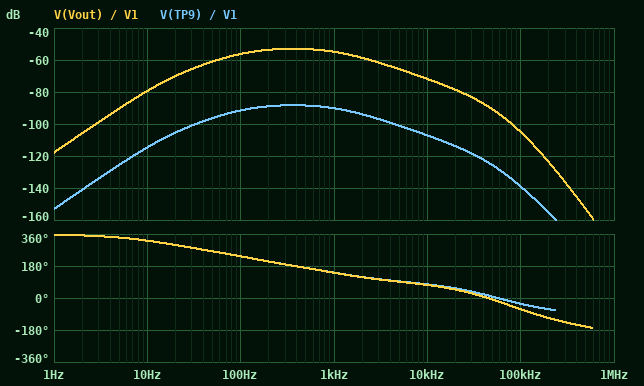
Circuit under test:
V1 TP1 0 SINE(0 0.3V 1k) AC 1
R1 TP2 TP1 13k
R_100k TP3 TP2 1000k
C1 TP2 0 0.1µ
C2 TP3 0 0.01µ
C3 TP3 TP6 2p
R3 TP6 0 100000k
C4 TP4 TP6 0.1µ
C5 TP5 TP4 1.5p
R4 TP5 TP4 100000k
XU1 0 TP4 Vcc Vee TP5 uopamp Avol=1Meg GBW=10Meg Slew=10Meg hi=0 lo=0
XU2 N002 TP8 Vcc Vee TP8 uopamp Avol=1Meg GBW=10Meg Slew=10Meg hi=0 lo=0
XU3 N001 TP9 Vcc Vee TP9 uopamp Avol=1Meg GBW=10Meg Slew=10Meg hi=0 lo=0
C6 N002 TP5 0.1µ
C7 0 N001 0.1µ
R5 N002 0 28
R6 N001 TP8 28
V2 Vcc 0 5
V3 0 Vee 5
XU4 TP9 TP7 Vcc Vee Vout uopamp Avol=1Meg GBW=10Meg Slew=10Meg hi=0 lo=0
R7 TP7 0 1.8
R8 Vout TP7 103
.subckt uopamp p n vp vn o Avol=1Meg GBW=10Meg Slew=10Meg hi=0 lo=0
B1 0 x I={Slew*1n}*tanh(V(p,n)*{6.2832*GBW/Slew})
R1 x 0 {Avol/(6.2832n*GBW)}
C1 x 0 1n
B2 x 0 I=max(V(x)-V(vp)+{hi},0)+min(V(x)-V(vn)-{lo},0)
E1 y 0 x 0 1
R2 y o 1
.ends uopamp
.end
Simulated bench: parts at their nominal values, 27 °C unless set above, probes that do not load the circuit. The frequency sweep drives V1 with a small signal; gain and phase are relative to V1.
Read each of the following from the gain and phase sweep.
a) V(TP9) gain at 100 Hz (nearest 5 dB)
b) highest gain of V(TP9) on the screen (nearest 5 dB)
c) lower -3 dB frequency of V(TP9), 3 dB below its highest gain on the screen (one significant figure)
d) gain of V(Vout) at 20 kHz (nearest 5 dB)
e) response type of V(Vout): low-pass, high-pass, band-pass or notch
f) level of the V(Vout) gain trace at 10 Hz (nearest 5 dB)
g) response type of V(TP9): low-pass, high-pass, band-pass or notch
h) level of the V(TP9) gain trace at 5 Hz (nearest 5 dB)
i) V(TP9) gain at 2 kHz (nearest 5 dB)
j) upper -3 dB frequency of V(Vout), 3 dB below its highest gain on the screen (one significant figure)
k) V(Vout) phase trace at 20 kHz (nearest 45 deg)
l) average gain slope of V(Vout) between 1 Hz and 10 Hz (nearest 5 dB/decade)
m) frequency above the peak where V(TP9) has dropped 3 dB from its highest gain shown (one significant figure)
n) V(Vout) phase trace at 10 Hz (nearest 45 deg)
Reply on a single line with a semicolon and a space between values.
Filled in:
-90 dB; -90 dB; 100 Hz; -80 dB; band-pass; -80 dB; band-pass; -125 dB; -95 dB; 1 kHz; 45 deg; 40 dB/decade; 1 kHz; 315 deg
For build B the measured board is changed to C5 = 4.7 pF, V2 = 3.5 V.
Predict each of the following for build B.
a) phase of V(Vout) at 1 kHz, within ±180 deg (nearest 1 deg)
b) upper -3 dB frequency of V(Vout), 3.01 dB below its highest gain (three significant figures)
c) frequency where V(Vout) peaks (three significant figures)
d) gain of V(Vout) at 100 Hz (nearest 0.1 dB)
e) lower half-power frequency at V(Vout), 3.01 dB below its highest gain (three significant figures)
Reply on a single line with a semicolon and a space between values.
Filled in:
114 deg; 543 Hz; 207 Hz; -56.5 dB; 79.7 Hz
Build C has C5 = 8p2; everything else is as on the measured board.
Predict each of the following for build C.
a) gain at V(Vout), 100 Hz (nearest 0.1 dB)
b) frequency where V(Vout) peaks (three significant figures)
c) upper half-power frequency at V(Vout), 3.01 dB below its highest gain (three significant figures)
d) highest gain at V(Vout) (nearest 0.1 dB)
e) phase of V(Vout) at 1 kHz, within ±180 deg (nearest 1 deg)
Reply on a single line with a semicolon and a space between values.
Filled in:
-57.2 dB; 157 Hz; 384 Hz; -56.4 dB; 107 deg
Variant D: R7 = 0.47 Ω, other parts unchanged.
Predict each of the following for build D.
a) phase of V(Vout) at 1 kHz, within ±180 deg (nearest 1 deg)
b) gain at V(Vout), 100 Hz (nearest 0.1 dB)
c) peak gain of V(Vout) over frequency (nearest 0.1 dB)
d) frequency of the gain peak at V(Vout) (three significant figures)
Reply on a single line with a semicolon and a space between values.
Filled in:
141 deg; -44.7 dB; -41.4 dB; 365 Hz
